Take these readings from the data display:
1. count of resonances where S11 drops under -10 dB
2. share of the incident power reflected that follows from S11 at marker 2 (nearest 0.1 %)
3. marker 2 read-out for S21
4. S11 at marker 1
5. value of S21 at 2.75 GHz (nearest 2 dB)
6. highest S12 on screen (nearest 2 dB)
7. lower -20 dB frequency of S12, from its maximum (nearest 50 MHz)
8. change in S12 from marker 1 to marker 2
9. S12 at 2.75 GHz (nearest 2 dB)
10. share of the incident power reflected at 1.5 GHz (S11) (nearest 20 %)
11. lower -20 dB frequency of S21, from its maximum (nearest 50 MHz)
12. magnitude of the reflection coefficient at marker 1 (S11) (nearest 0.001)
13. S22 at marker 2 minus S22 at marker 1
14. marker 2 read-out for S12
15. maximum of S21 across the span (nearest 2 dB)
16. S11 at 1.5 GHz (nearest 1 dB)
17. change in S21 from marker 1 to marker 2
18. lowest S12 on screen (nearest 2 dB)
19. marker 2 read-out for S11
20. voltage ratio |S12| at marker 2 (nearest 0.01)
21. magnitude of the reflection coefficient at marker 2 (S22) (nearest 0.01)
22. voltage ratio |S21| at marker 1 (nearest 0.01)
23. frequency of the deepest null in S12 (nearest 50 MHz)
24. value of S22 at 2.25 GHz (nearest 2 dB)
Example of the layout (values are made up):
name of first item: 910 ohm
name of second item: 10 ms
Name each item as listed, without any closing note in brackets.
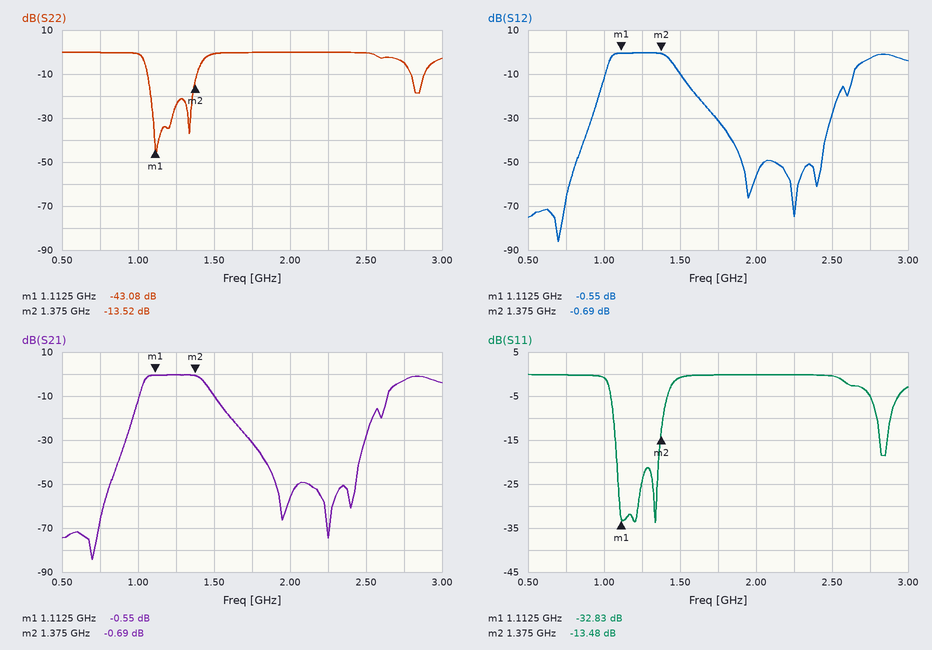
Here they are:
count of resonances where S11 drops under -10 dB: 3
share of the incident power reflected that follows from S11 at marker 2: 4.5 %
marker 2 read-out for S21: -0.69 dB
S11 at marker 1: -32.83 dB
value of S21 at 2.75 GHz: -2 dB
highest S12 on screen: 0 dB
lower -20 dB frequency of S12, from its maximum: 950 MHz
change in S12 from marker 1 to marker 2: -0.14 dB
S12 at 2.75 GHz: -2 dB
share of the incident power reflected at 1.5 GHz (S11): 80 %
lower -20 dB frequency of S21, from its maximum: 950 MHz
magnitude of the reflection coefficient at marker 1 (S11): 0.023
S22 at marker 2 minus S22 at marker 1: 29.56 dB
marker 2 read-out for S12: -0.69 dB
maximum of S21 across the span: 0 dB
S11 at 1.5 GHz: -1 dB
change in S21 from marker 1 to marker 2: -0.14 dB
lowest S12 on screen: -86 dB
marker 2 read-out for S11: -13.48 dB
voltage ratio |S12| at marker 2: 0.92
magnitude of the reflection coefficient at marker 2 (S22): 0.21
voltage ratio |S21| at marker 1: 0.94
frequency of the deepest null in S12: 700 MHz
value of S22 at 2.25 GHz: 0 dB
